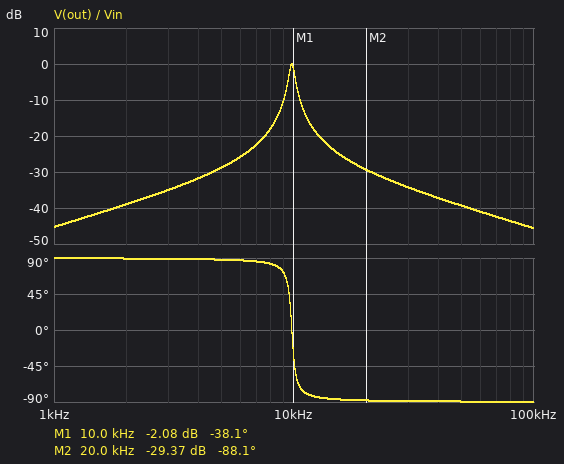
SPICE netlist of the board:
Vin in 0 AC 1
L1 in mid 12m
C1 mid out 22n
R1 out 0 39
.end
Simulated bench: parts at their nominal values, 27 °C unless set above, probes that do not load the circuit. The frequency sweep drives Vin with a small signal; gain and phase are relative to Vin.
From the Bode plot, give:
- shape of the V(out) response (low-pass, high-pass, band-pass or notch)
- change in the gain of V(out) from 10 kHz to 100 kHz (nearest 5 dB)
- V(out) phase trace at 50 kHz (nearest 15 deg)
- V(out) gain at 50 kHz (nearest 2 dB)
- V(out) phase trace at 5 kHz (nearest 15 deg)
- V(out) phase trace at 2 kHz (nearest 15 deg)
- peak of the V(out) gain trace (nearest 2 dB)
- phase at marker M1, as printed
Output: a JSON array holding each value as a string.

["band-pass", "-45 dB", "-90 deg", "-40 dB", "90 deg", "90 deg", "0 dB", "-38.1 deg"]
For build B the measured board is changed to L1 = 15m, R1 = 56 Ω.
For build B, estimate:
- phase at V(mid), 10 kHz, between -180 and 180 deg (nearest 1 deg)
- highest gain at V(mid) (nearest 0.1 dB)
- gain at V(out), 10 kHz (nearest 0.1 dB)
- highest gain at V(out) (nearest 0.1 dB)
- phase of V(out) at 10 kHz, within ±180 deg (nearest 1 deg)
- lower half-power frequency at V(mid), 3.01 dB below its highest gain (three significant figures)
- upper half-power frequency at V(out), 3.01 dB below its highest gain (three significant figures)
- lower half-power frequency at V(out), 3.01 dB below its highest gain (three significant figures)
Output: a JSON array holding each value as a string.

["-161 deg", "23.4 dB", "-12.1 dB", "0 dB", "-76 deg", "8.45 kHz", "9.06 kHz", "8.47 kHz"]
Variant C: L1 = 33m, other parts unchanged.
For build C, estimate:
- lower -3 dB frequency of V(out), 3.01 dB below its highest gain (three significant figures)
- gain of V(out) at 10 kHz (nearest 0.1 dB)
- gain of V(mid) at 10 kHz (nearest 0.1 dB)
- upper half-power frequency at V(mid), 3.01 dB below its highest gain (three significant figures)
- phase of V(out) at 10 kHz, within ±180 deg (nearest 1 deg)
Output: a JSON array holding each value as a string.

["5.81 kHz", "-30.8 dB", "-5.4 dB", "6.00 kHz", "-88 deg"]
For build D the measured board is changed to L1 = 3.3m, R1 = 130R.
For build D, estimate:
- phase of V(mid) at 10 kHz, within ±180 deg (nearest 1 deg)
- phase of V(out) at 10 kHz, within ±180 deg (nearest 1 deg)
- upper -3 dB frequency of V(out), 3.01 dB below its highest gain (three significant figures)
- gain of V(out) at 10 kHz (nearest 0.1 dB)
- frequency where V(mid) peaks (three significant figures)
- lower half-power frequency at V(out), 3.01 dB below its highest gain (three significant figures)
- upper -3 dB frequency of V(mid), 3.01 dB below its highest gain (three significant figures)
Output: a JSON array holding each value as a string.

["-4 deg", "76 deg", "22.1 kHz", "-12.2 dB", "18.2 kHz", "15.8 kHz", "21.2 kHz"]
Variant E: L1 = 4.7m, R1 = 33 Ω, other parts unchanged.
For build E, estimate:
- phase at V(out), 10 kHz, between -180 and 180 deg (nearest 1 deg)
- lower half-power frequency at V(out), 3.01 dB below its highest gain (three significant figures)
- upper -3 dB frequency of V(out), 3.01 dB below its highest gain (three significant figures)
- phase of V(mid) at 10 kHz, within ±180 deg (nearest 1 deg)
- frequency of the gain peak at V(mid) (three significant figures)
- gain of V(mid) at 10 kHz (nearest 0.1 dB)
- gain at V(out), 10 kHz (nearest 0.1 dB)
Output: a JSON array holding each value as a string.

["86 deg", "15.1 kHz", "16.2 kHz", "-2 deg", "15.6 kHz", "4.5 dB", "-22.3 dB"]
